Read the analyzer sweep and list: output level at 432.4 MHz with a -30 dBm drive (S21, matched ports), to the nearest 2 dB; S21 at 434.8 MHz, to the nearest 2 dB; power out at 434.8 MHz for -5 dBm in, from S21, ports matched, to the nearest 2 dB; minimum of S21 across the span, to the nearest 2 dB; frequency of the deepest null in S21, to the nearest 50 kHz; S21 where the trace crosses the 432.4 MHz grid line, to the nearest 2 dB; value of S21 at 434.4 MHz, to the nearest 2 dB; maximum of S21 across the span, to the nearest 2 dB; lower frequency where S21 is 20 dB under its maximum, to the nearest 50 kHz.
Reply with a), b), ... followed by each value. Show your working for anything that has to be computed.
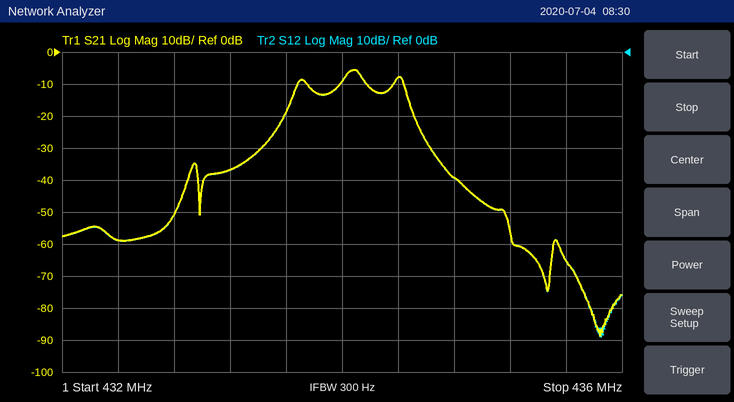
a) -30 dBm + (-58 dB) = -88 dBm
b) -40 dB
c) -5 dBm + (-40 dB) = -44 dBm
d) -88 dB
e) 435.85 MHz
f) -58 dB
g) -8 dB
h) -6 dB
i) 433.50 MHz
